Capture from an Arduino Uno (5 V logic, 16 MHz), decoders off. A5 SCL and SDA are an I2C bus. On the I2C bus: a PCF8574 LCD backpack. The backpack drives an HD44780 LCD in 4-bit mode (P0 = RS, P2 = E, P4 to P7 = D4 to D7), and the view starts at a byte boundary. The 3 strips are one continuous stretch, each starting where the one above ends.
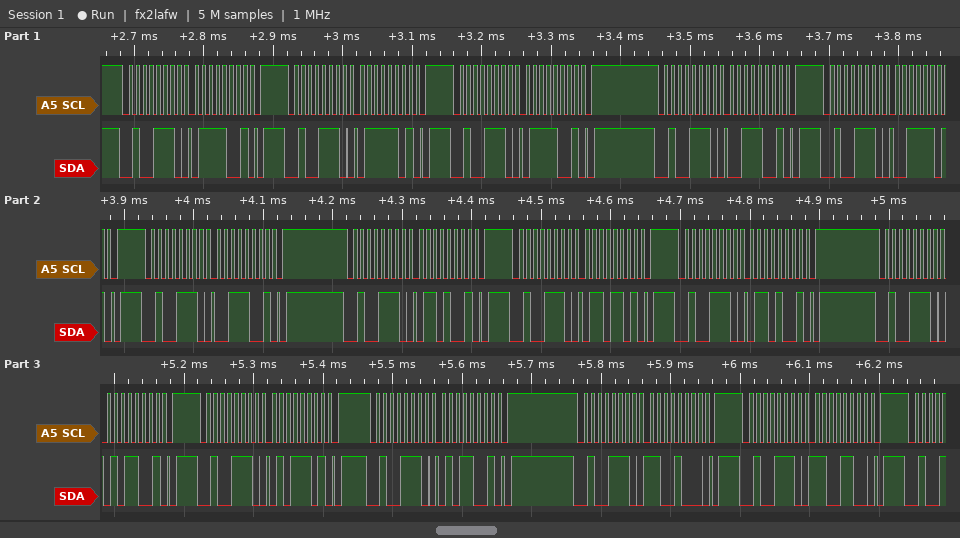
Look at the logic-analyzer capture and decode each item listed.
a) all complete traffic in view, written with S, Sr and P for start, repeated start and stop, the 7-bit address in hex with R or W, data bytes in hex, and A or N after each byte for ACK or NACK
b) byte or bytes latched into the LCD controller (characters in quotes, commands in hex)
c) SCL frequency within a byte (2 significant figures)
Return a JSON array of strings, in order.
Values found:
["S 27W A 79 A P S 27W A 7D A P S 27W A 79 A P S 27W A 39 A P S 27W A 3D A P S 27W A 39 A P S 27W A 69 A P S 27W A 6D A P S 27W A 69 A P S 27W A 59 A P S 27W A 5D A P S 27W A 59 A P S 27W A C8 A P S 27W A CC A P", "'s' 'e'", "100 kHz"]
